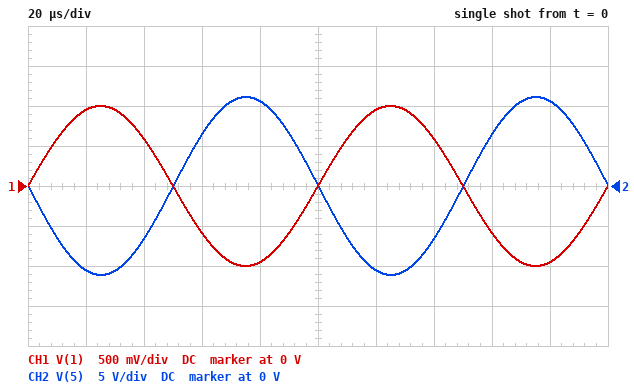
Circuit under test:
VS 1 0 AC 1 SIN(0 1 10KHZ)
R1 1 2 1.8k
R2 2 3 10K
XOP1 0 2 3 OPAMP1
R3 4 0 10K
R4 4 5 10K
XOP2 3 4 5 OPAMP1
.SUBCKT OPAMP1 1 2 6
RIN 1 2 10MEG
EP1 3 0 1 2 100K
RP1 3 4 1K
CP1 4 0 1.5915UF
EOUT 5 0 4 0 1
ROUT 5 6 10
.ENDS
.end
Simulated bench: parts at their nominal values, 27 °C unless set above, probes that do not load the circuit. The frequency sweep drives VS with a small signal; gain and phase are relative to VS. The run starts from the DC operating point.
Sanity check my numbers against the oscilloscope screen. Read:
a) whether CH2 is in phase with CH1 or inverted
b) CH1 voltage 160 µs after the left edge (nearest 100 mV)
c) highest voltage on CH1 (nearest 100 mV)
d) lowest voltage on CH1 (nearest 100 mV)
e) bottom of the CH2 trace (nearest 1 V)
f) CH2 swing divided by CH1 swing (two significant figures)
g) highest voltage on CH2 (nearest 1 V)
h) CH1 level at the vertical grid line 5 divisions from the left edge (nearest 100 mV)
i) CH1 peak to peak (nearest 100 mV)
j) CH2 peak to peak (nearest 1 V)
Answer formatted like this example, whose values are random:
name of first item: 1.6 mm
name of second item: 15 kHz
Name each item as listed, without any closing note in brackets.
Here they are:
whether CH2 is in phase with CH1 or inverted: inverted
CH1 voltage 160 µs after the left edge: -600 mV
highest voltage on CH1: 1.0 V
lowest voltage on CH1: -1.0 V
bottom of the CH2 trace: -11 V
CH2 swing divided by CH1 swing: 11
highest voltage on CH2: 11 V
CH1 level at the vertical grid line 5 divisions from the left edge: 0 V
CH1 peak to peak: 2.0 V
CH2 peak to peak: 22 V
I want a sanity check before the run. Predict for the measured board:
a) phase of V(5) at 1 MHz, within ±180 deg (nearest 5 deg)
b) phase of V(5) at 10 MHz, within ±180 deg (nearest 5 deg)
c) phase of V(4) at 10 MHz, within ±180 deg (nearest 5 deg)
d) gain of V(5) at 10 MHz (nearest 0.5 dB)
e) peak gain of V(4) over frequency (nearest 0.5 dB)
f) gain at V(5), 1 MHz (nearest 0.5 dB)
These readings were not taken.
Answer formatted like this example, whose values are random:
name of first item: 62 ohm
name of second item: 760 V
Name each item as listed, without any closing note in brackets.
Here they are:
phase of V(5) at 1 MHz, within ±180 deg: 135 deg
phase of V(5) at 10 MHz, within ±180 deg: 35 deg
phase of V(4) at 10 MHz, within ±180 deg: 35 deg
gain of V(5) at 10 MHz: -2.5 dB
peak gain of V(4) over frequency: 15.0 dB
gain at V(5), 1 MHz: 19.0 dB
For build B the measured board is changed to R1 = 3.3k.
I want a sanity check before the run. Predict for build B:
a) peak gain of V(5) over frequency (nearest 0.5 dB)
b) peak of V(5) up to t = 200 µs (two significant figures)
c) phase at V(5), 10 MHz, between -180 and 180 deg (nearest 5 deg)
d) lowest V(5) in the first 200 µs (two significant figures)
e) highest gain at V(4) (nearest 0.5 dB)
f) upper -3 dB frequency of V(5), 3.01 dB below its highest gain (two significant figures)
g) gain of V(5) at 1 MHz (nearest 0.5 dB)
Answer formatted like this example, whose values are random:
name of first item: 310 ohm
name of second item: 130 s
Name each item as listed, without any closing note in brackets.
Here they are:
peak gain of V(5) over frequency: 15.5 dB
peak of V(5) up to t = 200 µs: 6.1 V
phase at V(5), 10 MHz, between -180 and 180 deg: 40 deg
lowest V(5) in the first 200 µs: -6.1 V
highest gain at V(4): 9.5 dB
upper -3 dB frequency of V(5), 3.01 dB below its highest gain: 2.1 MHz
gain of V(5) at 1 MHz: 15.0 dB
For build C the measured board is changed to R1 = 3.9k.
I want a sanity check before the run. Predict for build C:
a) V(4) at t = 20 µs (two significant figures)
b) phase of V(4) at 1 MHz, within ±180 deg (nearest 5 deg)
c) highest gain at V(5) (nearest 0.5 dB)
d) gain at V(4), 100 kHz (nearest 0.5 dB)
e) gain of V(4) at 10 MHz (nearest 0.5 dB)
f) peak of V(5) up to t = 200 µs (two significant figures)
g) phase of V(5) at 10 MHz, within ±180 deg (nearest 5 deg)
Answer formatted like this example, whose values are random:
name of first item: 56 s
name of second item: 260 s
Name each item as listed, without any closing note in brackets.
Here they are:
V(4) at t = 20 µs: -2.4 V
phase of V(4) at 1 MHz, within ±180 deg: 150 deg
highest gain at V(5): 14.0 dB
gain at V(4), 100 kHz: 8.0 dB
gain of V(4) at 10 MHz: -10.0 dB
peak of V(5) up to t = 200 µs: 5.1 V
phase of V(5) at 10 MHz, within ±180 deg: 40 deg
